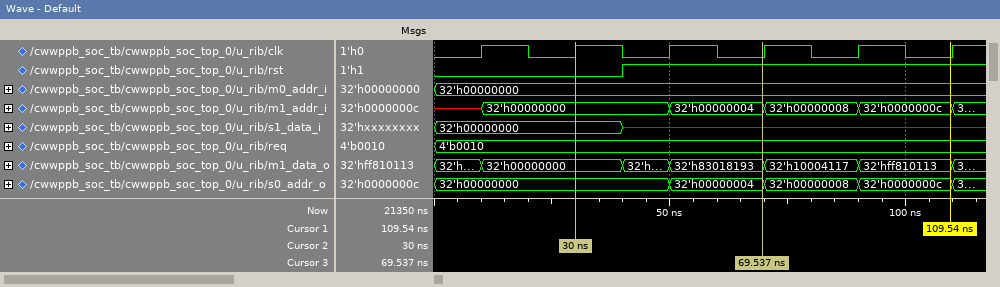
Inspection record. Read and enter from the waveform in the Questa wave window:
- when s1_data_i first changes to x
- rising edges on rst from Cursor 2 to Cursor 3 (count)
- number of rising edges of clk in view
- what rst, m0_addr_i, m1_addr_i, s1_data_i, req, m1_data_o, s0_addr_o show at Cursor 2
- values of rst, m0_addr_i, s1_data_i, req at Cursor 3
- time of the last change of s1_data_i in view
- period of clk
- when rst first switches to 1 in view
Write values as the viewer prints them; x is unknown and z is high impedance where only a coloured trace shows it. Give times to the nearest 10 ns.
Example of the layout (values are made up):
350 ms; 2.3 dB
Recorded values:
40 ns; 1; 6; rst=0, m0_addr_i=32'h00000000, m1_addr_i=32'h00000000, s1_data_i=32'h00000000, req=4'b0010, m1_data_o=32'h00000000, s0_addr_o=32'h00000000; rst=1, m0_addr_i=32'h00000000, s1_data_i=x, req=4'b0010; 40 ns; 20 ns; 40 ns
